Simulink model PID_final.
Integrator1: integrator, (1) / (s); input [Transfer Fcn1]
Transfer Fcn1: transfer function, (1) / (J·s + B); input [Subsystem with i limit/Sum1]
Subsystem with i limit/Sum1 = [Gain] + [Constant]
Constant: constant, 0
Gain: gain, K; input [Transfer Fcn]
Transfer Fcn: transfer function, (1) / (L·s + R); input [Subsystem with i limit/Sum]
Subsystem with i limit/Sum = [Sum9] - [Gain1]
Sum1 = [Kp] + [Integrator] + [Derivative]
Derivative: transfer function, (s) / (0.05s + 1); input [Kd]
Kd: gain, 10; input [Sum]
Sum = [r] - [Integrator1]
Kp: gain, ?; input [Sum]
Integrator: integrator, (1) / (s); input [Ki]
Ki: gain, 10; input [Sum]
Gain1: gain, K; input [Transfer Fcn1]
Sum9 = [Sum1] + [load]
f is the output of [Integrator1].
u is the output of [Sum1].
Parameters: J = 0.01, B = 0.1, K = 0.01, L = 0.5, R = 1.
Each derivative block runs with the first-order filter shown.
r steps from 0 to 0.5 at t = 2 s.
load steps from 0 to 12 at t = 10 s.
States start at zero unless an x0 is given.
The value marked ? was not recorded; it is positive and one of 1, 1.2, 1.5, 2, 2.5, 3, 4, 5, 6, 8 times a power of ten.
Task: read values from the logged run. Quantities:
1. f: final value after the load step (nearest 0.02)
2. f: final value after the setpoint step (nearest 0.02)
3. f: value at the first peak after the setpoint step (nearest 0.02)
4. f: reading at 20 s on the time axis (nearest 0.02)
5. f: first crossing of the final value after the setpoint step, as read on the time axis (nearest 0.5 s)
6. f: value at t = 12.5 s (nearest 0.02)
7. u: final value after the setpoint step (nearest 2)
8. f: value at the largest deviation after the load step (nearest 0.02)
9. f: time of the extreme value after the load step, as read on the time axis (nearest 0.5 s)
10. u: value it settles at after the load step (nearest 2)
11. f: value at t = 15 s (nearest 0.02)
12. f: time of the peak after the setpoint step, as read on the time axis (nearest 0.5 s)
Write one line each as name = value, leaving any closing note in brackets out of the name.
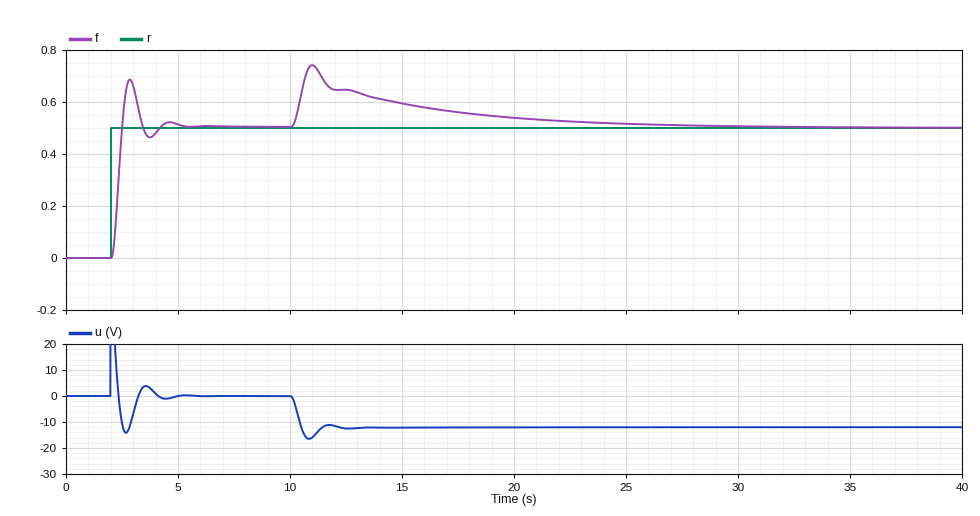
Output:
f: final value after the load step = 0.50
f: final value after the setpoint step = 0.50
f: value at the first peak after the setpoint step = 0.68
f: reading at 20 s on the time axis = 0.54
f: first crossing of the final value after the setpoint step, as read on the time axis = 2.5 s
f: value at t = 12.5 s = 0.64
u: final value after the setpoint step = 0
f: value at the largest deviation after the load step = 0.74
f: time of the extreme value after the load step, as read on the time axis = 11.0 s
u: value it settles at after the load step = -12
f: value at t = 15 s = 0.60
f: time of the peak after the setpoint step, as read on the time axis = 3.0 s
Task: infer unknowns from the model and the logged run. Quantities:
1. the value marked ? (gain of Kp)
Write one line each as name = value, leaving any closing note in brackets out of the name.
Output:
the value marked ? = 60
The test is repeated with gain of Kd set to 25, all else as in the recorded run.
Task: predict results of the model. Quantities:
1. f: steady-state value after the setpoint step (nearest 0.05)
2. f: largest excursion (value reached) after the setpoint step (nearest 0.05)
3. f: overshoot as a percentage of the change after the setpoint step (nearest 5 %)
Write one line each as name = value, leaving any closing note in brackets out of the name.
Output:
f: steady-state value after the setpoint step = 0.50
f: largest excursion (value reached) after the setpoint step = 0.60
f: overshoot as a percentage of the change after the setpoint step = 20 %
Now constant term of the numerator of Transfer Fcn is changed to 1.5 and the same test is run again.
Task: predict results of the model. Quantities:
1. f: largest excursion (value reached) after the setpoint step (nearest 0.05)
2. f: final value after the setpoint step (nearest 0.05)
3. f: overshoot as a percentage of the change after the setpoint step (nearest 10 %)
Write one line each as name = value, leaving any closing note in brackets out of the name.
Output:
f: largest excursion (value reached) after the setpoint step = 0.75
f: final value after the setpoint step = 0.50
f: overshoot as a percentage of the change after the setpoint step = 50 %
